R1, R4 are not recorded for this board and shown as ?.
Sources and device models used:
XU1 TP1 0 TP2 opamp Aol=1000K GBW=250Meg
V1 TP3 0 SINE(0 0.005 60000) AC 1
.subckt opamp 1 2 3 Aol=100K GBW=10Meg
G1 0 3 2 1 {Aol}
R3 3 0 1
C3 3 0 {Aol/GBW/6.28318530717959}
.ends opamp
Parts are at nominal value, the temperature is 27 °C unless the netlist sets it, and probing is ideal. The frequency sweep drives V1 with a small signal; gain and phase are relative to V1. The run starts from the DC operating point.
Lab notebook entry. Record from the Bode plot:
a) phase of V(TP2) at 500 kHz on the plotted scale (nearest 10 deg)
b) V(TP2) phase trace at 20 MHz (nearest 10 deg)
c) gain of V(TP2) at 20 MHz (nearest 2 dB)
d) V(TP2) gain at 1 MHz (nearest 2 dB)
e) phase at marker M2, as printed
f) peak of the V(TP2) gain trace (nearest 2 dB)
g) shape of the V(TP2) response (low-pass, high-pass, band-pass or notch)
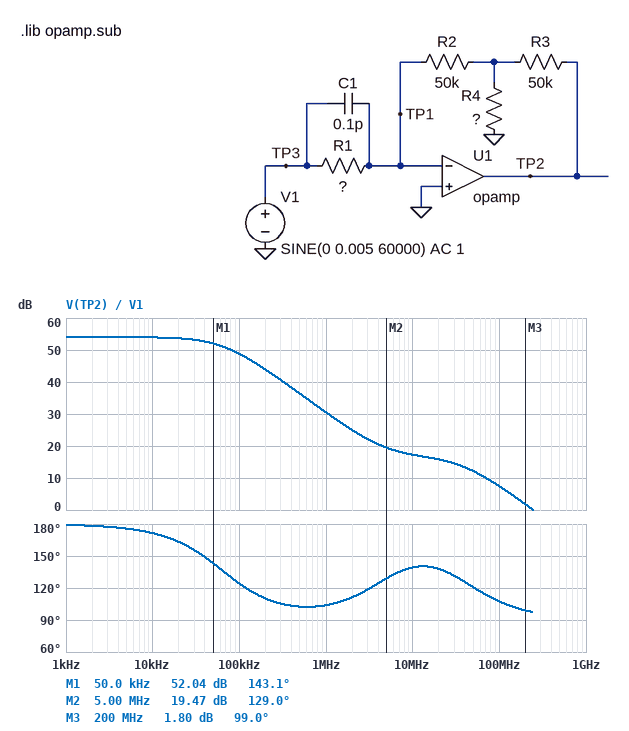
100 deg
140 deg
16 dB
30 dB
129.0 deg
54 dB
low-pass
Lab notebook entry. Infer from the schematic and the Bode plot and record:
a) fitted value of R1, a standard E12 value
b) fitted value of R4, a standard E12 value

330 kΩ
15 Ω
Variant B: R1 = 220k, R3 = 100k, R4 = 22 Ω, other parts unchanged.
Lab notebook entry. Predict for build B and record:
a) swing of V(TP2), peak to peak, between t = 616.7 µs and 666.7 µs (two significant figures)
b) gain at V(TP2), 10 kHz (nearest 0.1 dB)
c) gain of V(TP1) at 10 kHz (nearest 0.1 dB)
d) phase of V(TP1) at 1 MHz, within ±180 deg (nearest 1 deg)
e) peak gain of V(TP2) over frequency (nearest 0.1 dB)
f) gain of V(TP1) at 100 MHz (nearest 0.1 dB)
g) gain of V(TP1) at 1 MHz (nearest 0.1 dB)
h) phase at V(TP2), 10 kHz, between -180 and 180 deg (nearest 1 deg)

6.2 V
60.0 dB
-27.9 dB
9 deg
60.2 dB
-0.6 dB
-14.6 dB
168 deg
